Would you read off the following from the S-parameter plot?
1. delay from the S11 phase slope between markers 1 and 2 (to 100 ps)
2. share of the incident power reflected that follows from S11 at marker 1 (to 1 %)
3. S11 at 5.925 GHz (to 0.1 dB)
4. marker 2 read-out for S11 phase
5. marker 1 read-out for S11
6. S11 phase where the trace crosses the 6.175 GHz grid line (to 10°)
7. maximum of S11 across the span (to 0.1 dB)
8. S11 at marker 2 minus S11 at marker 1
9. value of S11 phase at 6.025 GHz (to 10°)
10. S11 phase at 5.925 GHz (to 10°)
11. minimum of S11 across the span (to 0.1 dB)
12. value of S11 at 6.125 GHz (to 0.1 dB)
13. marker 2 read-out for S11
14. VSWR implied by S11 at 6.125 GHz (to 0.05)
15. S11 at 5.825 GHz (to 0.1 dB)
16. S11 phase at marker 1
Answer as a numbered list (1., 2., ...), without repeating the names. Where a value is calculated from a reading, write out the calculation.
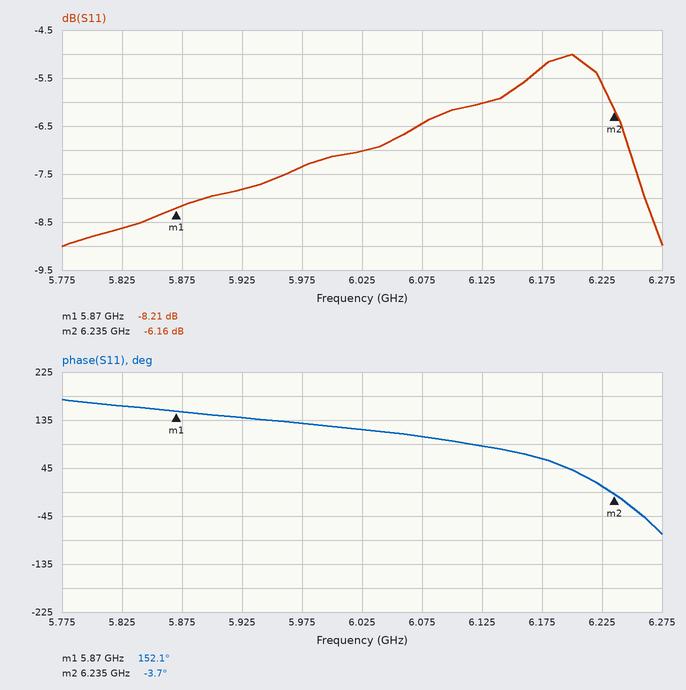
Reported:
1. −(-3.7° − (152.1°))/(360° × 365 MHz) ≈ 1.2 ns
2. 10^(-8.21/10) ≈ 15 %
3. -7.8 dB
4. -3.7°
5. -8.21 dB
6. 60°
7. -5.0 dB
8. -6.16 − (-8.21) = 2.05 dB
9. 120°
10. 140°
11. -9.0 dB
12. -6.0 dB
13. -6.16 dB
14. |Γ| = 10^(-6/20) = 0.5012; VSWR = (1 + 0.5012)/(1 − 0.5012) ≈ 3.01, so 3.00 to the nearest 0.05
15. -8.6 dB
16. 152.1°
